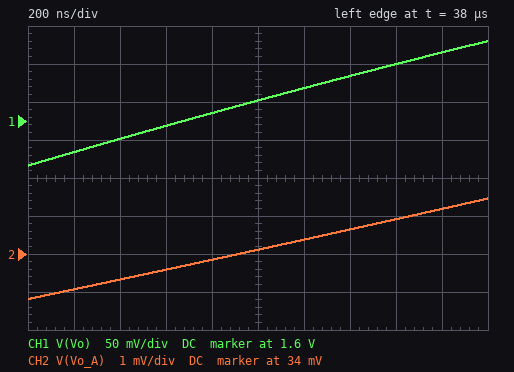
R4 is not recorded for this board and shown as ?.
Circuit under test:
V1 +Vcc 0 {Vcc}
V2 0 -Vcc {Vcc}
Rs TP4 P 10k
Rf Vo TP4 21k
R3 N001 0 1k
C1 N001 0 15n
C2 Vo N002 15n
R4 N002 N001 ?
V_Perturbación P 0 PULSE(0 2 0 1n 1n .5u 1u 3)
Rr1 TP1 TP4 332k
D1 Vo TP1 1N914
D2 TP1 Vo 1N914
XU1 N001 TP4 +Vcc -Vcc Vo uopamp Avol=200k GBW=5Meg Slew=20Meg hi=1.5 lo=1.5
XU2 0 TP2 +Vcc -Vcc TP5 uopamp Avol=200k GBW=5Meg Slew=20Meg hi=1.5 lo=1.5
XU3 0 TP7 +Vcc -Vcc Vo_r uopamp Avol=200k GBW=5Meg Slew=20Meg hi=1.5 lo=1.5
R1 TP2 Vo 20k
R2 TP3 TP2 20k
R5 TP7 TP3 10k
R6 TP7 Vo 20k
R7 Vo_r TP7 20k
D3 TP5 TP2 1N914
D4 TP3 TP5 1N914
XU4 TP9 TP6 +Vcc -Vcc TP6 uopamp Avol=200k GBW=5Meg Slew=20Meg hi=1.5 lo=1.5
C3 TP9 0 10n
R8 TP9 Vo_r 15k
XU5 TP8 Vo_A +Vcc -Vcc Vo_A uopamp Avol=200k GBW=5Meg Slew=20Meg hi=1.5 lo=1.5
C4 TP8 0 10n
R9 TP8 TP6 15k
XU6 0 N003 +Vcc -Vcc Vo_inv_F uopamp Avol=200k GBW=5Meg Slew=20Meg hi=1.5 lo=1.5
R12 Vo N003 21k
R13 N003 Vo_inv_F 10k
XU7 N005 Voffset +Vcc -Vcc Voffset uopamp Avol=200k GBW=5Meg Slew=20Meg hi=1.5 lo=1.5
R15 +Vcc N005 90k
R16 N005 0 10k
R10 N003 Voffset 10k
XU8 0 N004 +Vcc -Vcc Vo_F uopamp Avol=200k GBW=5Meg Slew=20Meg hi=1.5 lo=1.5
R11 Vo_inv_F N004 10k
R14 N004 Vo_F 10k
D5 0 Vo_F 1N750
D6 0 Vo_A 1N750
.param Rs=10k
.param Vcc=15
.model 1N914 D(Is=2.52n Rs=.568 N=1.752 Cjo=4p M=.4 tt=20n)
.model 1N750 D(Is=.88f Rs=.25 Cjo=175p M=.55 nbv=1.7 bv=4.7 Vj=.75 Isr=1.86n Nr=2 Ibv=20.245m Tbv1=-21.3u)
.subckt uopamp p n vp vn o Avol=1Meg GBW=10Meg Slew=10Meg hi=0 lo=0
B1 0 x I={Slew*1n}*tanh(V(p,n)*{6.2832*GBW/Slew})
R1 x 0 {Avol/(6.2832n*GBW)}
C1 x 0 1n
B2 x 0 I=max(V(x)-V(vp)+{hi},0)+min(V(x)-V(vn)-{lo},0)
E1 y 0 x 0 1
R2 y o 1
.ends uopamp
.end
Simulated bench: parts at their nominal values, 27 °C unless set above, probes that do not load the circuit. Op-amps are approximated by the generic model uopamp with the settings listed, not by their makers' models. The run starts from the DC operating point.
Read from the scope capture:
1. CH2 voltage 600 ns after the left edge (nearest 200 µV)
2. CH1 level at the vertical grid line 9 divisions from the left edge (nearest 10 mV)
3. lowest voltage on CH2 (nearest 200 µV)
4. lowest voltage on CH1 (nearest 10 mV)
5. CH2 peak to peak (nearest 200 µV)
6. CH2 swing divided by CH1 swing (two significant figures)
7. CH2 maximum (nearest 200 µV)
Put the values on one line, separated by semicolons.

33.6 mV; 1.69 V; 32.8 mV; 1.54 V; 2.6 mV; 0.016; 35.4 mV
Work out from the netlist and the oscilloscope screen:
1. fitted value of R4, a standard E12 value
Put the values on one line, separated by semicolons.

820 Ω
